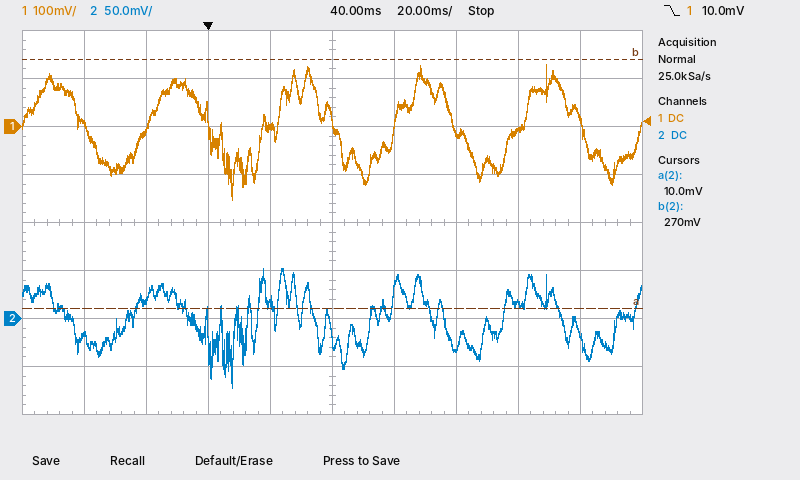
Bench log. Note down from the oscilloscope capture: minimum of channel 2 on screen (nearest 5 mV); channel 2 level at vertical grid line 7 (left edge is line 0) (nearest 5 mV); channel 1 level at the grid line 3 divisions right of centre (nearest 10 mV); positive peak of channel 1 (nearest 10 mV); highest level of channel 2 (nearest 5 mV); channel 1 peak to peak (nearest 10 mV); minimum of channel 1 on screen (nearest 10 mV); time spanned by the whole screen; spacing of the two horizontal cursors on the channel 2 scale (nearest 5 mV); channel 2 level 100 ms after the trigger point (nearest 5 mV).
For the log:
-70 mV
-30 mV
-10 mV
130 mV
50 mV
280 mV
-150 mV
200 ms
260 mV
15 mV
